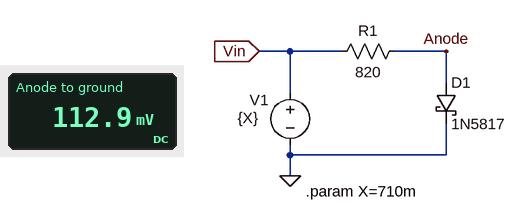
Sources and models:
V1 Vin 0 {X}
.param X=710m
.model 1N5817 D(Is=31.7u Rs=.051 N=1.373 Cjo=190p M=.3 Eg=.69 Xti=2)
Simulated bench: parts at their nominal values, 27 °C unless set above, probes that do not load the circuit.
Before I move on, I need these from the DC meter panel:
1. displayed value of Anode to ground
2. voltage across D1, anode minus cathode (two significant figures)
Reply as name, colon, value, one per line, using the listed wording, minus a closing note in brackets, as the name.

displayed value of Anode to ground: 112.9 mV
voltage across D1, anode minus cathode: 110 mV
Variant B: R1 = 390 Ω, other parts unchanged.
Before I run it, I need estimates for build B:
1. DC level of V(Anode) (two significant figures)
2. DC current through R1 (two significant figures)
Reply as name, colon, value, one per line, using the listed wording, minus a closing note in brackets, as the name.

DC level of V(Anode): 140 mV
DC current through R1: 1.5 mA
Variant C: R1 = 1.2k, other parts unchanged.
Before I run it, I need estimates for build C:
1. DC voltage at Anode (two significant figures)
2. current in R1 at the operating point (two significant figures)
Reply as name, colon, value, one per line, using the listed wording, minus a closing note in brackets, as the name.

DC voltage at Anode: 100 mV
current in R1 at the operating point: 510 µA
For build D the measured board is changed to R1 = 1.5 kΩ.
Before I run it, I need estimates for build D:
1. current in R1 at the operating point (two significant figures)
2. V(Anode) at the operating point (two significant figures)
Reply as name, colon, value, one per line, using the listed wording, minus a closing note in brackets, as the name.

current in R1 at the operating point: 410 µA
V(Anode) at the operating point: 94 mV
